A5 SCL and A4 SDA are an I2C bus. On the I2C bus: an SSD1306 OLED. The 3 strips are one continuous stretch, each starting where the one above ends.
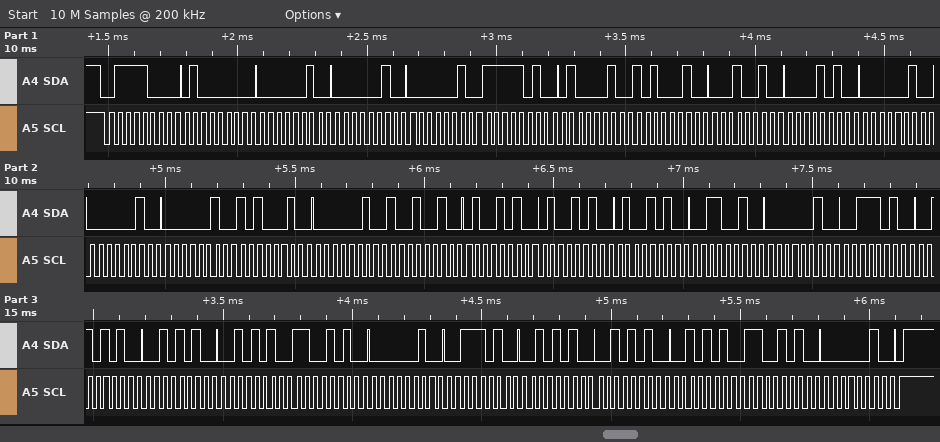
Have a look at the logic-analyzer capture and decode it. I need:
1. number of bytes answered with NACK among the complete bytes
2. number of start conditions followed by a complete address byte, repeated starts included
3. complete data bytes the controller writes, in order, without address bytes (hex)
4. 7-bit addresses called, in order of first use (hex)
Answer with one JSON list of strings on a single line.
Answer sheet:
["0", "1", "40 02 02 02 FA 42 A2 12 0A 02 02 02 A2 02 92 4A 4A 4A 32 02 3A 2A 2A 2A CA 02 3A 2A 2A 2A CA 02", "0x3C"]
